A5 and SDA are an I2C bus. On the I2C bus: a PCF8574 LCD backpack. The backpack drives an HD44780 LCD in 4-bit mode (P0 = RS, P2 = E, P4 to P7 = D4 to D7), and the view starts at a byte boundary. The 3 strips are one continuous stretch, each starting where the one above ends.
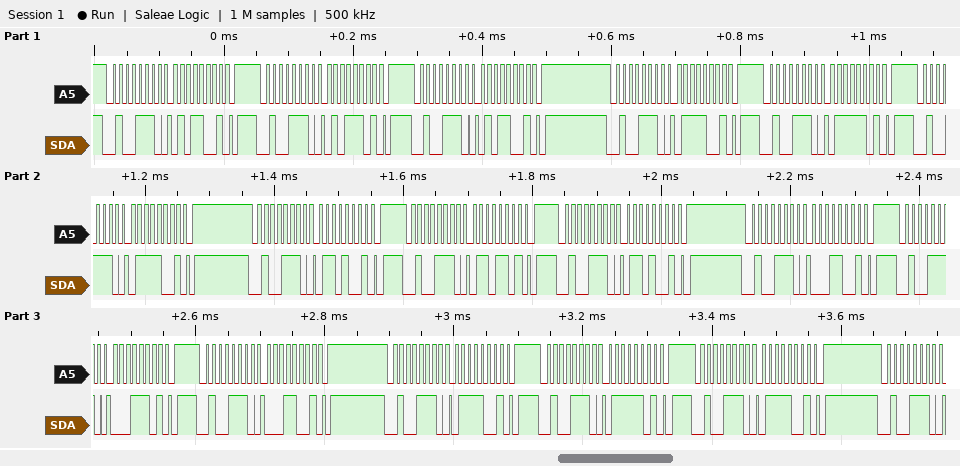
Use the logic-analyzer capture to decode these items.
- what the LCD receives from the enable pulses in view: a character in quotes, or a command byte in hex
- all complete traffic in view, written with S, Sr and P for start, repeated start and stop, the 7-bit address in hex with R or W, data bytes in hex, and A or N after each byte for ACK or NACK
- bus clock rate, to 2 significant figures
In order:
'W' 'a'
S 27W A 59 A P S 27W A 5D A P S 27W A 59 A P S 27W A 79 A P S 27W A 7D A P S 27W A 79 A P S 27W A 69 A P S 27W A 6D A P S 27W A 69 A P S 27W A 19 A P S 27W A 1D A P S 27W A 19 A P S 27W A 79 A P S 27W A 7D A P S 27W A 79 A P S 27W A
100 kHz
